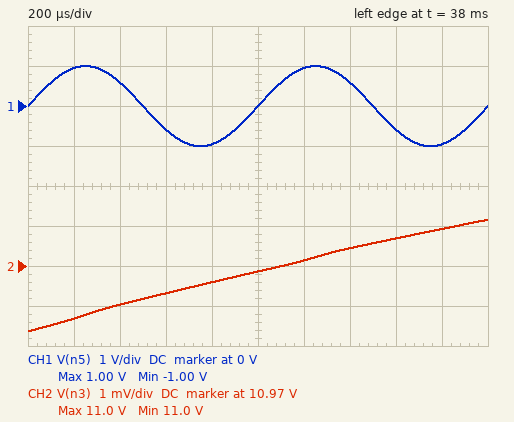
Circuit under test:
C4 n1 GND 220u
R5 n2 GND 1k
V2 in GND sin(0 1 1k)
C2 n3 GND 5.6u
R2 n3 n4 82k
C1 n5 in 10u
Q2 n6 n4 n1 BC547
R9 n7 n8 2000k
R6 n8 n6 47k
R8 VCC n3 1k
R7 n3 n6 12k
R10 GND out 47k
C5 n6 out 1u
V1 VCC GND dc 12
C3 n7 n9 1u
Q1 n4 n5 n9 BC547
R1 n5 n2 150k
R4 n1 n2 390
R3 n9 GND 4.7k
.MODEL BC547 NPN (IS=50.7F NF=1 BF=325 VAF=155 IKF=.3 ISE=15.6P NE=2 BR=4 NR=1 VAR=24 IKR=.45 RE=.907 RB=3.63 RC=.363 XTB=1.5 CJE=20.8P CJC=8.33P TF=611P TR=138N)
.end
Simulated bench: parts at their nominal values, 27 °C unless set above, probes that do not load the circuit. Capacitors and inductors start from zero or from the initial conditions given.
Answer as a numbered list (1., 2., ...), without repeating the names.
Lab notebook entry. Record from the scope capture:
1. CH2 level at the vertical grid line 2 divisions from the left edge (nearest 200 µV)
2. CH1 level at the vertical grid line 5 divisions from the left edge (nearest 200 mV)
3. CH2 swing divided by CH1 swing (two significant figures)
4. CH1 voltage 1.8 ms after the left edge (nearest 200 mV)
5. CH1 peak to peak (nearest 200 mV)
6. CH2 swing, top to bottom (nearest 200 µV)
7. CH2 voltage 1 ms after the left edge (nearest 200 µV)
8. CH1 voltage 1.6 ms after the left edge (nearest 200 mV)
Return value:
1. 10.9680 V
2. 0 V
3. 0.0014
4. -1.0 V
5. 2.0 V
6. 2.8 mV
7. 10.9688 V
8. -600 mV
